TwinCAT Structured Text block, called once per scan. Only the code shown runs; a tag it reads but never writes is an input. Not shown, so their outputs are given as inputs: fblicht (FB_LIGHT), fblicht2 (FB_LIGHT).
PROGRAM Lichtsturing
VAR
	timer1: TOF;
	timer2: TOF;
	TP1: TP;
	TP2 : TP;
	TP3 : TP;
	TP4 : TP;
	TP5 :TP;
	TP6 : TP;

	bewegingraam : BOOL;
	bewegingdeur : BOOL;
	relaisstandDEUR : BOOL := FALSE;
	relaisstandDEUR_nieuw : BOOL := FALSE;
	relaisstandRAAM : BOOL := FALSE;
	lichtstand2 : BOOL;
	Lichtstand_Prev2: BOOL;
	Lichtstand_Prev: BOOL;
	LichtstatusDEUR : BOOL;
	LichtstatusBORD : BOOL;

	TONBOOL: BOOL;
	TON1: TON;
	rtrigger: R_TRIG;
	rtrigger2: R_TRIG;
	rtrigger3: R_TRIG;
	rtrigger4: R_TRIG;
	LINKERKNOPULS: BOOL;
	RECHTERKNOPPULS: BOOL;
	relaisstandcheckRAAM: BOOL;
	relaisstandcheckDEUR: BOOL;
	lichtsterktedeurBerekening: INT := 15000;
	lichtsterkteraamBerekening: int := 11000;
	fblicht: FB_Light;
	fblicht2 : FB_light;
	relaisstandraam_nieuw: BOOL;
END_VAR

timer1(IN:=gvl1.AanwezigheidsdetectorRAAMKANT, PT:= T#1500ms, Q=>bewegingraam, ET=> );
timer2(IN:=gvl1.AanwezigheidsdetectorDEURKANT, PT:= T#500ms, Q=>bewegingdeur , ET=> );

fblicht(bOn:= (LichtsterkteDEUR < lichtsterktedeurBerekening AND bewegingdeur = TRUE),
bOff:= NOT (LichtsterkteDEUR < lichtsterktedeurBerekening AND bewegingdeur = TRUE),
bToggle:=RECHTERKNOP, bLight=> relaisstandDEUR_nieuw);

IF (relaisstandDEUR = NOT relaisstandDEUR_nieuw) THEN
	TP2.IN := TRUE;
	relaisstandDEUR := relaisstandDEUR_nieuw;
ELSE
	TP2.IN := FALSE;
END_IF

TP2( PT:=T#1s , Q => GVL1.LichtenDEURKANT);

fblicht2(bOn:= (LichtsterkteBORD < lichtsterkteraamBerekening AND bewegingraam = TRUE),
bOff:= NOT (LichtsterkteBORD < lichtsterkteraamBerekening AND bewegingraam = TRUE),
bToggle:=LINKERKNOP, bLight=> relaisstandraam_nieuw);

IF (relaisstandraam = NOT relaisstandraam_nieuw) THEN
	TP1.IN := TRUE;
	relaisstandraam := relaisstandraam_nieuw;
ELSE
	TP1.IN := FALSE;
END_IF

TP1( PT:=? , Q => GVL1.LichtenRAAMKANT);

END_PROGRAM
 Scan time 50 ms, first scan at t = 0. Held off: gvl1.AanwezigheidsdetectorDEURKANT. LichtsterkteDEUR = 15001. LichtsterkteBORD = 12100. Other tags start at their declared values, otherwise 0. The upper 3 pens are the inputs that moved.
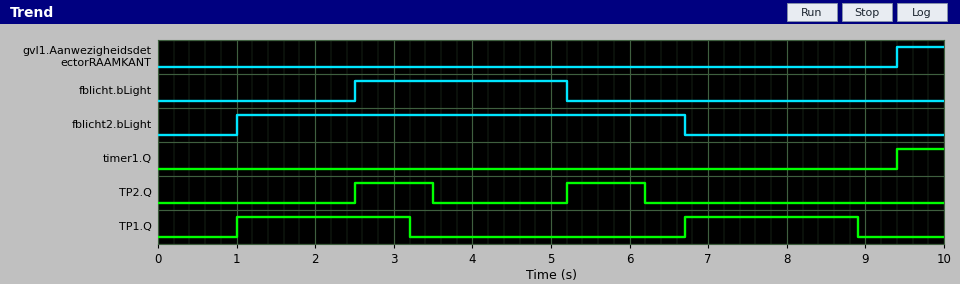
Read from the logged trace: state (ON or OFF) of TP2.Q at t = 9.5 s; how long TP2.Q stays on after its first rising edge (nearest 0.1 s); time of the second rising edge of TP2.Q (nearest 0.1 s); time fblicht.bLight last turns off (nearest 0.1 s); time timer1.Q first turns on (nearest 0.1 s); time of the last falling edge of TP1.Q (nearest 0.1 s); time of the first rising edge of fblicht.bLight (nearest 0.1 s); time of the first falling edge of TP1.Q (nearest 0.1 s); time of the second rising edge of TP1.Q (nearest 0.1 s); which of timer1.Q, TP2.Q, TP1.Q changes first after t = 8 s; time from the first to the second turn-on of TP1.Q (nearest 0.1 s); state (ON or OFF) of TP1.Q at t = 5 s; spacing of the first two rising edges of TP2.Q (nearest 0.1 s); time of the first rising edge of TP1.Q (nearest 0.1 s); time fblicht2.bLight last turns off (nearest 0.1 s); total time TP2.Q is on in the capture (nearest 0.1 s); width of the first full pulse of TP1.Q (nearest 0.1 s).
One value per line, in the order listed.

OFF
1.0 s
5.2 s
5.2 s
9.4 s
8.9 s
2.5 s
3.2 s
6.7 s
TP1.Q
5.7 s
OFF
2.7 s
1.0 s
6.7 s
2.0 s
2.2 s
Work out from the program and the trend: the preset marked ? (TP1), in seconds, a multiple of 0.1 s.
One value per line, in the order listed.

2.2 s
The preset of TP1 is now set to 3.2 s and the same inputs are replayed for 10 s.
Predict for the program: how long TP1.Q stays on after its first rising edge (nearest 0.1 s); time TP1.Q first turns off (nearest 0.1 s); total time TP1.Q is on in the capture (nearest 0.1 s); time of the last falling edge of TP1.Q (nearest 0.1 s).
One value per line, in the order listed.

3.2 s
4.2 s
6.4 s
9.9 s
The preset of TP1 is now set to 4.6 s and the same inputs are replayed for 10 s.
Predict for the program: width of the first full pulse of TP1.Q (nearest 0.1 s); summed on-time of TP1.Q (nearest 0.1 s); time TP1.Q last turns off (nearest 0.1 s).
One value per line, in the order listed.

4.6 s
7.9 s
5.6 s
